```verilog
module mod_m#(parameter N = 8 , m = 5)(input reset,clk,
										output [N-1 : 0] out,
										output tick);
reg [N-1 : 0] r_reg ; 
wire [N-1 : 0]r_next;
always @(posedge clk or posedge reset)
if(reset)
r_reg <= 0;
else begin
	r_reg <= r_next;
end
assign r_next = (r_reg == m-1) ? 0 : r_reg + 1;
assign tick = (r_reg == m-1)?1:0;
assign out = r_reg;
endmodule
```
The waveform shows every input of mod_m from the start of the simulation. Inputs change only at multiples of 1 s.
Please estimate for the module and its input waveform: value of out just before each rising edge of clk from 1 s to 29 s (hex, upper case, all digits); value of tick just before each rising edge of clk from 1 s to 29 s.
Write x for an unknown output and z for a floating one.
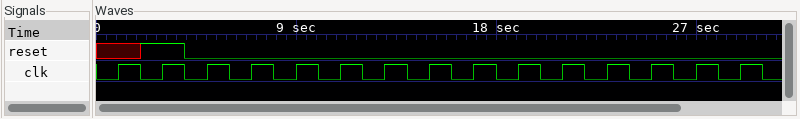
x, 00, 00, 01, 02, 03, 04, 00, 01, 02, 03, 04, 00, 01, 02
x 0 0 0 0 0 1 0 0 0 0 1 0 0 0
